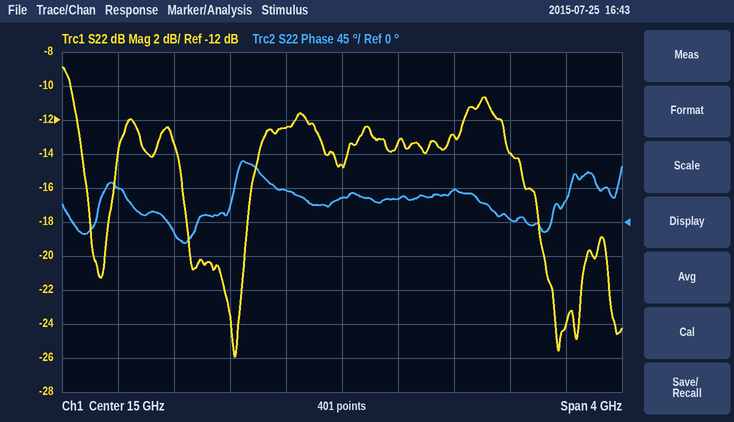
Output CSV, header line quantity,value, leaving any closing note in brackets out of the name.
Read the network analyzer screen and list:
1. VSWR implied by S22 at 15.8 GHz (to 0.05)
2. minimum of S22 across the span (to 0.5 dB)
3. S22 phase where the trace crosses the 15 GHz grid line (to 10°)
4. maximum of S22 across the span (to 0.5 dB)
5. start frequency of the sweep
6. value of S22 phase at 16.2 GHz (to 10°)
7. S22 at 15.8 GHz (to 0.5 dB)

quantity,value
VSWR implied by S22 at 15.8 GHz,1.60
minimum of S22 across the span,-26.0 dB
S22 phase where the trace crosses the 15 GHz grid line,30°
maximum of S22 across the span,-9.0 dB
start frequency of the sweep,13 GHz
value of S22 phase at 16.2 GHz,0°
S22 at 15.8 GHz,-13.0 dB
